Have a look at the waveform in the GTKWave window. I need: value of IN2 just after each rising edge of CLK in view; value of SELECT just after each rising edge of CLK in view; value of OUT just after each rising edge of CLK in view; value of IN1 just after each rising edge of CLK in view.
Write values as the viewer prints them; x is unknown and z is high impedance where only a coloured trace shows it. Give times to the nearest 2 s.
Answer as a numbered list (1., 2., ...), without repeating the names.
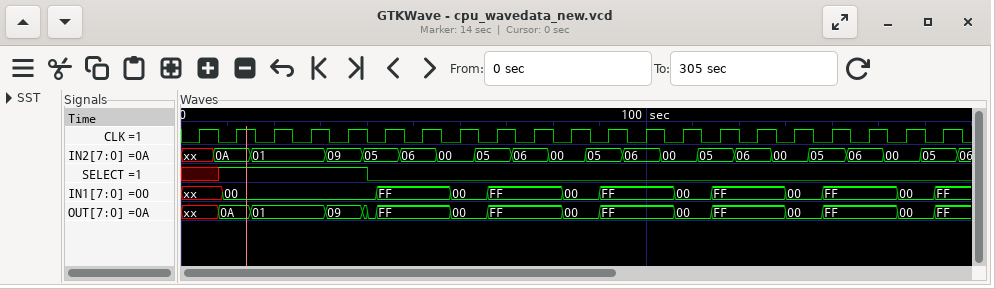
1. xx, 0A, 01, 01, 09, 05, 06, 00, 05, 06, 00, 05, 06, 00, 05, 06, 00, 05, 06, 00, 05
2. x 1 1 1 1 0 0 0 0 0 0 0 0 0 0 0 0 0 0 0 0
3. xx, 0A, 01, 01, 09, FF, FF, 00, FF, FF, 00, FF, FF, 00, FF, FF, 00, FF, FF, 00, FF
4. xx, 00, 00, 00, 00, FF, FF, 00, FF, FF, 00, FF, FF, 00, FF, FF, 00, FF, FF, 00, FF
